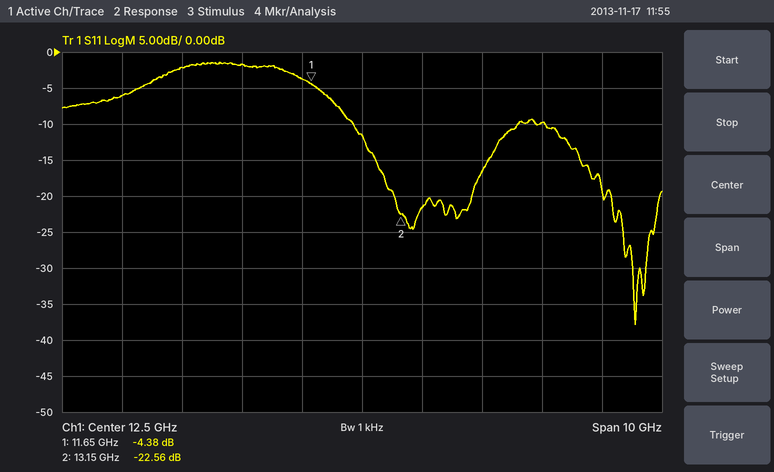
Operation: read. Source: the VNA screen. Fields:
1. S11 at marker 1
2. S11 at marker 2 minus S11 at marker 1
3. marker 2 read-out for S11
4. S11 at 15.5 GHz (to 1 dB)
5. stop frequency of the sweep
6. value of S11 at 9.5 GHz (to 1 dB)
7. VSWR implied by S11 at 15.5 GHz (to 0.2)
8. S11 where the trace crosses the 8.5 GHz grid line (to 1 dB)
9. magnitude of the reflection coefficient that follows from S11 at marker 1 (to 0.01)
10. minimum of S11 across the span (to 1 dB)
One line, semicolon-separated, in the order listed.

-4.38 dB; -18.18 dB; -22.56 dB; -10 dB; 17.5 GHz; -2 dB; 2.0; -6 dB; 0.60; -38 dB
